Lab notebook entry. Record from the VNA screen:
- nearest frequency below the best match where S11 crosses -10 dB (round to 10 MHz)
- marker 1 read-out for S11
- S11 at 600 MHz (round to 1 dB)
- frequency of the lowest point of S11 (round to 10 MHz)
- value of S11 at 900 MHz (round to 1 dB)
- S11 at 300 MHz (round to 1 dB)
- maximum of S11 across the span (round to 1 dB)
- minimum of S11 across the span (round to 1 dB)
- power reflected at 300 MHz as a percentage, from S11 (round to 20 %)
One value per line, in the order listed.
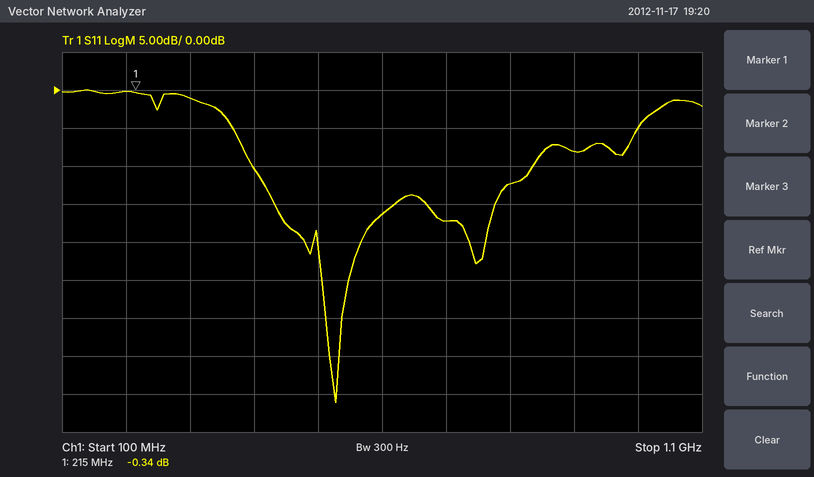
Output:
400 MHz
-0.34 dB
-16 dB
530 MHz
-8 dB
-1 dB
0 dB
-41 dB
80 %
